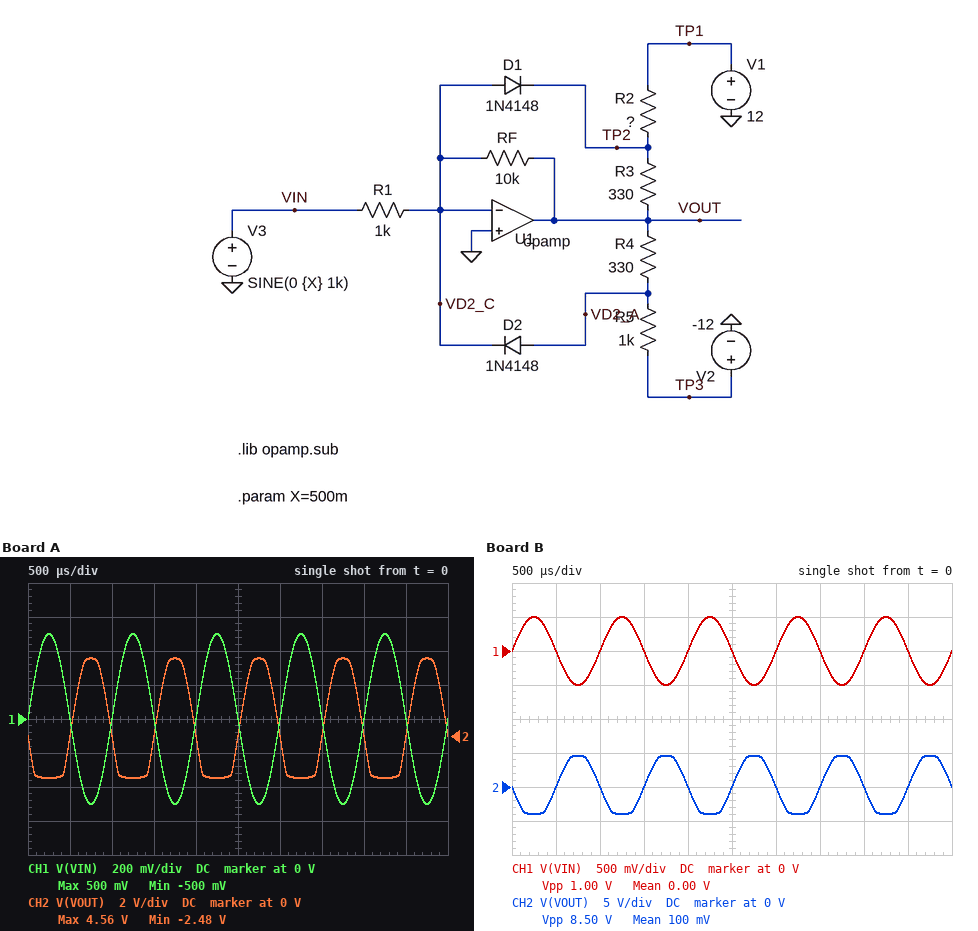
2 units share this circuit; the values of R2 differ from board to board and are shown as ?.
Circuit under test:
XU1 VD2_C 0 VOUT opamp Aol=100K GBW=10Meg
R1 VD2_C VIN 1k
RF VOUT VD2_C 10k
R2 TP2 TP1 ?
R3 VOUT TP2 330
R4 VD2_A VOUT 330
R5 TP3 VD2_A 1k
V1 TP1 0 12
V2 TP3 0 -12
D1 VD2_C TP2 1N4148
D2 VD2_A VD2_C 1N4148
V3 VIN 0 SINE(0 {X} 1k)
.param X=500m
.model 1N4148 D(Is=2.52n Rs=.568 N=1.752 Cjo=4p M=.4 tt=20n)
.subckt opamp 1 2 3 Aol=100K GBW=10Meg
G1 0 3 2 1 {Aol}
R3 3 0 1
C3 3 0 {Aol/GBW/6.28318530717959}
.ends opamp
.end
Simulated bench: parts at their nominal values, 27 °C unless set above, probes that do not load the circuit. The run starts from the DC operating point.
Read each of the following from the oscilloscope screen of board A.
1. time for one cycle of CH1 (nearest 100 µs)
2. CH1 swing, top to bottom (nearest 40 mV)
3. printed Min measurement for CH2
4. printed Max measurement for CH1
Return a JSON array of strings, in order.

["1.0 ms", "1.00 V", "-2.48 V", "500 mV"]
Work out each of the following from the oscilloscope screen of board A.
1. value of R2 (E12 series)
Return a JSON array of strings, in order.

["2.2 kΩ"]
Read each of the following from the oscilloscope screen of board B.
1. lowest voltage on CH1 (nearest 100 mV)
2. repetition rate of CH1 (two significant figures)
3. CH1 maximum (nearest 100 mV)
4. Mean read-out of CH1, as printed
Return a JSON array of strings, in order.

["-500 mV", "1.0 kHz", "500 mV", "0.00 V"]
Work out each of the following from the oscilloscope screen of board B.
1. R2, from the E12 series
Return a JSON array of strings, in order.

["1.2 kΩ"]
